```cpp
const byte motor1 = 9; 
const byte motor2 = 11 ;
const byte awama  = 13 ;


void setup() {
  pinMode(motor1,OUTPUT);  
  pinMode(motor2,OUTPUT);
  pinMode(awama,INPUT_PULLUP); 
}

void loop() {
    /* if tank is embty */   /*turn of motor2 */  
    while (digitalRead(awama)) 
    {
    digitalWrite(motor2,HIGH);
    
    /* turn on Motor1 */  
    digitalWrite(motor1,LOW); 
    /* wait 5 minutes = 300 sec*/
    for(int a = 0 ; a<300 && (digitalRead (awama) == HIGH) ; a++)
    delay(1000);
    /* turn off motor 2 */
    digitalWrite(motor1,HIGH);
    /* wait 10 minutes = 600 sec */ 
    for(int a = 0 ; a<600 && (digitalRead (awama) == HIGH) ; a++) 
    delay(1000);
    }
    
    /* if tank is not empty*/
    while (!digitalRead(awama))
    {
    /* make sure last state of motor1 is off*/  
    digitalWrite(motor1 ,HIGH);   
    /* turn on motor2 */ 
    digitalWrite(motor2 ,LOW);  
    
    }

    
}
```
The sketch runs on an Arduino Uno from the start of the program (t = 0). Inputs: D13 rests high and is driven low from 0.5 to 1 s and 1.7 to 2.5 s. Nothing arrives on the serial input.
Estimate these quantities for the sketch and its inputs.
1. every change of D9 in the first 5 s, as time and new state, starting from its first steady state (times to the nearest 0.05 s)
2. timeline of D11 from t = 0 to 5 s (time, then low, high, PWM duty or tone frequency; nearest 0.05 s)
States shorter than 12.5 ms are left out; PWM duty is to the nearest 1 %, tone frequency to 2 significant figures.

0 s low; 2 s high; 2.5 s low
0 s high; 2 s low; 2.5 s high
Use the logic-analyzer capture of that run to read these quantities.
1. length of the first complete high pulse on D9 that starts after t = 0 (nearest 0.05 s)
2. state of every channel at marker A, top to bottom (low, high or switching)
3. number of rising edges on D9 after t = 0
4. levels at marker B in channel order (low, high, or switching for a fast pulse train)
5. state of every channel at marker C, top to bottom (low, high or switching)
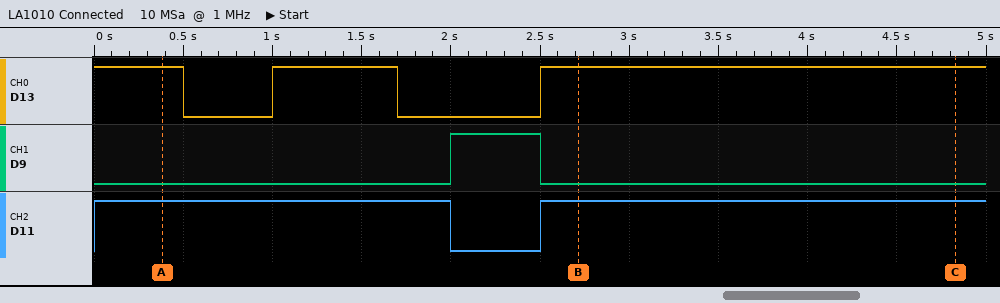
0.50 s
D13 high, D9 low, D11 high
1
D13 high, D9 low, D11 high
D13 high, D9 low, D11 high
